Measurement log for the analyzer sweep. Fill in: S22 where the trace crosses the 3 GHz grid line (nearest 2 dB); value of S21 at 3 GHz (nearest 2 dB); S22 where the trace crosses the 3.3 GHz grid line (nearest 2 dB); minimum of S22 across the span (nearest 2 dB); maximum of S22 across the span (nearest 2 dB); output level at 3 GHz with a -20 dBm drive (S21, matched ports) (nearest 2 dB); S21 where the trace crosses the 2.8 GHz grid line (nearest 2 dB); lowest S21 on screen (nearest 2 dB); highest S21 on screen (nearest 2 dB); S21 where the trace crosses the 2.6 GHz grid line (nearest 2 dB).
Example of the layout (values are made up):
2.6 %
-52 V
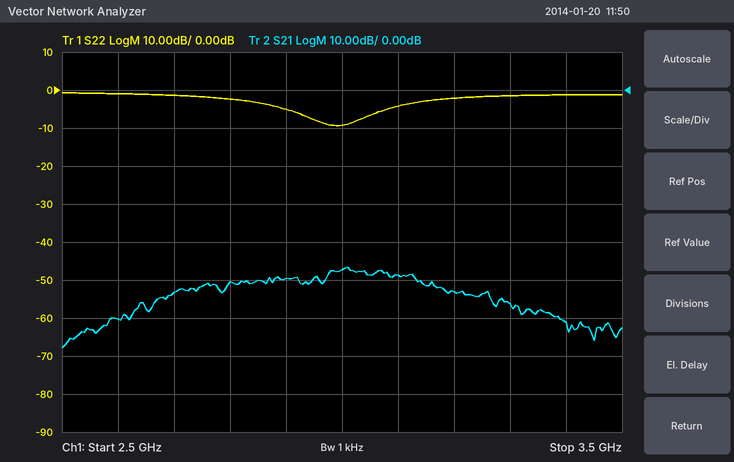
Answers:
-10 dB
-48 dB
-2 dB
-10 dB
0 dB
-68 dBm
-50 dB
-68 dB
-46 dB
-60 dB
